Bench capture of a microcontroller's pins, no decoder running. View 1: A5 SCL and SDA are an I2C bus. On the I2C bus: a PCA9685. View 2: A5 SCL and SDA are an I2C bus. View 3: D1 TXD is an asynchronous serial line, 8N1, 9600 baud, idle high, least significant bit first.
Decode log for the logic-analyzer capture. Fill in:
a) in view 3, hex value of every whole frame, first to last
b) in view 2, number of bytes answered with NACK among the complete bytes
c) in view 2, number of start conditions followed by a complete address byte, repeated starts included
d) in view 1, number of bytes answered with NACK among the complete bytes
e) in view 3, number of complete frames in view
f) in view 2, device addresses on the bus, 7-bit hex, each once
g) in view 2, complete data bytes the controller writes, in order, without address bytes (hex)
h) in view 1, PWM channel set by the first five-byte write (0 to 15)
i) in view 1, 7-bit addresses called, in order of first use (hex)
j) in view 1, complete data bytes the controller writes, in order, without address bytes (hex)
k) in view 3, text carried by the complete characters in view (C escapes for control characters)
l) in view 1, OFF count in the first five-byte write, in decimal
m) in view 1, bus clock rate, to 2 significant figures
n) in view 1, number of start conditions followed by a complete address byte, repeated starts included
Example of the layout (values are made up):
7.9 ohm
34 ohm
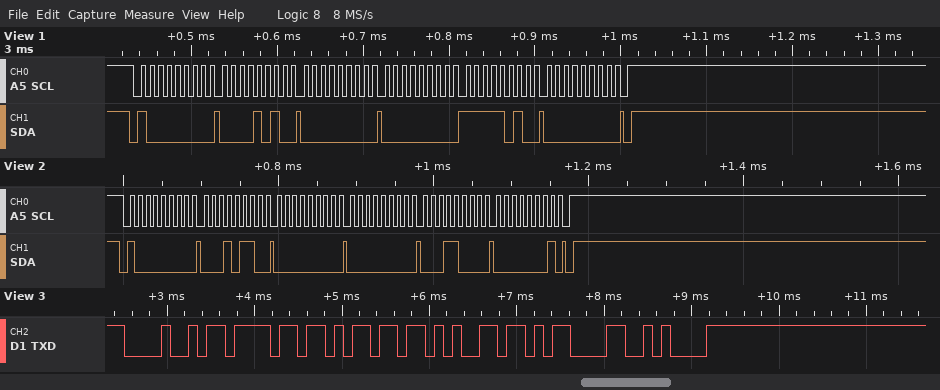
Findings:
0x48 0x6F 0x6D 0x65 0x0D 0x0A
0
1
0
6
0x40
16 00 00 18 01
1
0x40
0A 00 00 FA 00
"Home\r\n"
250
100 kHz
1
